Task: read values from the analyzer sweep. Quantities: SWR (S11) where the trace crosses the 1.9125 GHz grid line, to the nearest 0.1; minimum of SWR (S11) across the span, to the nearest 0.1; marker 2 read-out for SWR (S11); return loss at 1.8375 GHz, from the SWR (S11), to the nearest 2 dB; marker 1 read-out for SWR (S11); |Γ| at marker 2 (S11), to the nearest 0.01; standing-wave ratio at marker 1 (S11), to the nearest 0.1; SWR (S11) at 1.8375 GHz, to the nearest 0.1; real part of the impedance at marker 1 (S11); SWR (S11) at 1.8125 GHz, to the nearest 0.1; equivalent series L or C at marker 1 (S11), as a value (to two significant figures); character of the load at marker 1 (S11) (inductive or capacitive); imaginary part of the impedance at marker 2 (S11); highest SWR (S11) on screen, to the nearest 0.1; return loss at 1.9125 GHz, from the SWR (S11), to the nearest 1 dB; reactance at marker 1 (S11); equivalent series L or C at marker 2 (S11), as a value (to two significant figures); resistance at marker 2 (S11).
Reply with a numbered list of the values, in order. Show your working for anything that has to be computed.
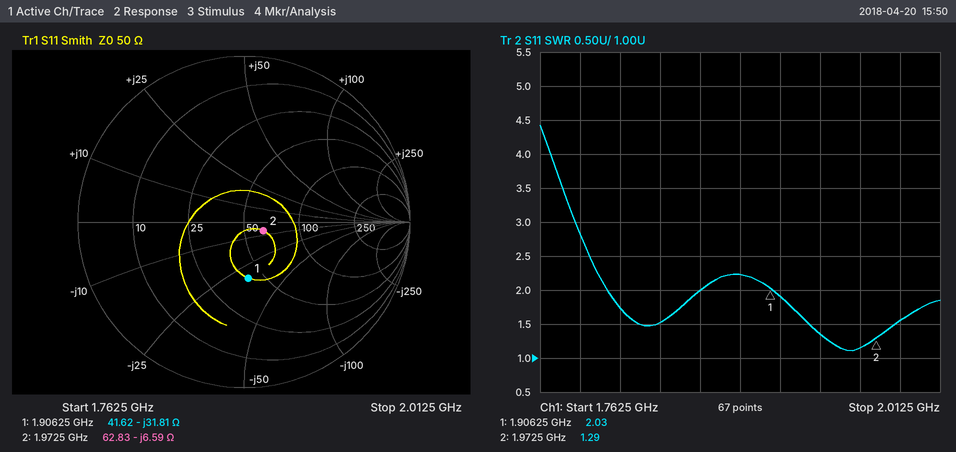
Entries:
1. 1.9
2. 1.1
3. 1.29
4. −20 log10((1.5 − 1)/(1.5 + 1)) ≈ 14 dB
5. 2.03
6. 0.13
7. 2.0
8. 1.5
9. 41.62 Ω
10. 1.7
11. C = 1/(2π × 1.90625 GHz × 31.81 Ω) ≈ 2.6 pF
12. capacitive
13. -6.59 Ω
14. 4.4
15. −20 log10((1.9 − 1)/(1.9 + 1)) ≈ 10 dB
16. -31.81 Ω
17. C = 1/(2π × 1.9725 GHz × 6.59 Ω) ≈ 12 pF
18. 62.83 Ω
